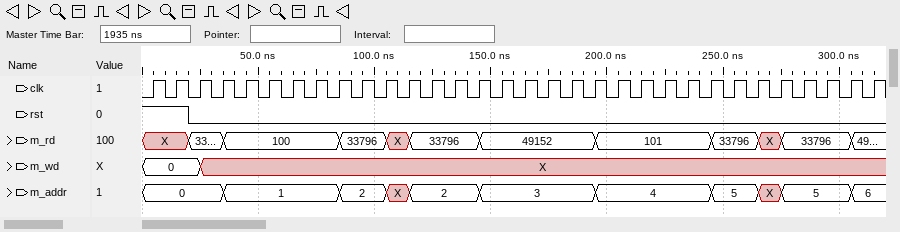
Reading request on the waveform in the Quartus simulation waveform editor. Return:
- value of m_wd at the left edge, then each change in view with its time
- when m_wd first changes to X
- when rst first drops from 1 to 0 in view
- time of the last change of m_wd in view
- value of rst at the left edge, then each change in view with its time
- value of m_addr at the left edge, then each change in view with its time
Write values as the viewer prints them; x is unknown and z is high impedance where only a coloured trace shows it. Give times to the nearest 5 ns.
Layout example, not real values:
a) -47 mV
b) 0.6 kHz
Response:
a) 0, X at 25 ns
b) 25 ns
c) 20 ns
d) 25 ns
e) 1, 0 at 20 ns
f) 0, 1 at 35 ns, 2 at 85 ns, X at 105 ns, 2 at 115 ns, 3 at 145 ns, 4 at 195 ns, 5 at 245 ns, X at 265 ns, 5 at 275 ns, 6 at 305 ns
